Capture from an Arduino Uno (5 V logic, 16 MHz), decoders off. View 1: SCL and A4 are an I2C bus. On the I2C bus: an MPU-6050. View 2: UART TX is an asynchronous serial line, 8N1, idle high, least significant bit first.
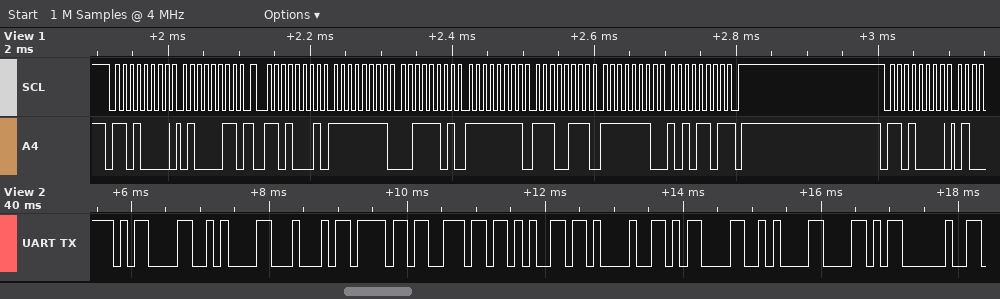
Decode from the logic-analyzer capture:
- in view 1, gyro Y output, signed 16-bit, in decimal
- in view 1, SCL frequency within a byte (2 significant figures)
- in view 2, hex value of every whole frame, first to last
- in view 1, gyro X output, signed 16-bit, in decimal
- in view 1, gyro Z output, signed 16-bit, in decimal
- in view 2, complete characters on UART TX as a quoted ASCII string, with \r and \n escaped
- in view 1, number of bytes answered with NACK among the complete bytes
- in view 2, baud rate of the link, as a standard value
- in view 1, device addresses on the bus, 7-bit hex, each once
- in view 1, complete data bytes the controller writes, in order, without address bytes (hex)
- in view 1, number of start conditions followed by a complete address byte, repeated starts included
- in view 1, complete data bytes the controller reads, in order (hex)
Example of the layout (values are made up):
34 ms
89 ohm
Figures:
-25
100 kHz
0D 0A 44 6F 6E 65 21 0D 0A 58 20
-195
-339
"\r\nDone!\r\nX "
1
9600 baud
0x68
43
3
FF 3D FF E7 FE AD
